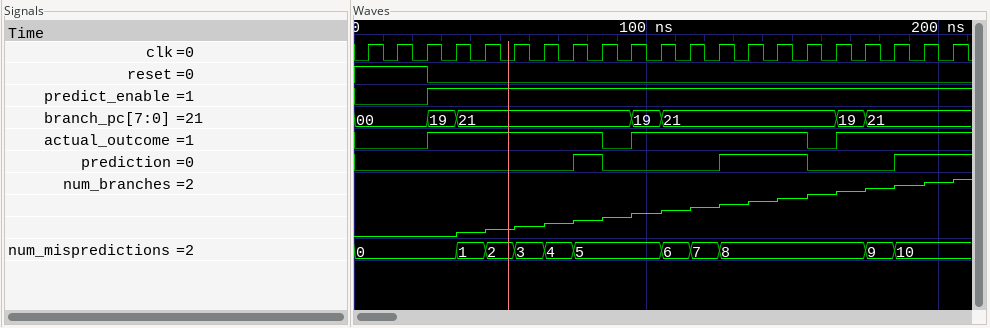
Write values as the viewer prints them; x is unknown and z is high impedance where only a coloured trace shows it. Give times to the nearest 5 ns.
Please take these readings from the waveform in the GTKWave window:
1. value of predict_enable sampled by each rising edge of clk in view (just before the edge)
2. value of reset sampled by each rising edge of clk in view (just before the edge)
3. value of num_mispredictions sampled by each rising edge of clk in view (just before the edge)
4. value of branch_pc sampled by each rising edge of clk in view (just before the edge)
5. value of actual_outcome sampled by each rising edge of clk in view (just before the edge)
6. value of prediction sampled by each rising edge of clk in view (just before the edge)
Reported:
0 0 0 1 1 1 1 1 1 1 1 1 1 1 1 1 1 1 1 1 1
1 1 1 0 0 0 0 0 0 0 0 0 0 0 0 0 0 0 0 0 0
0, 0, 0, 0, 1, 2, 3, 4, 5, 5, 5, 6, 7, 8, 8, 8, 8, 8, 9, 10, 10
00, 00, 00, 19, 21, 21, 21, 21, 21, 21, 19, 21, 21, 21, 21, 21, 21, 19, 21, 21, 21
0 0 0 1 1 1 1 1 1 0 1 1 1 1 1 1 0 1 1 1 1
0 0 0 0 0 0 0 0 1 0 0 0 0 1 1 1 0 0 0 1 1
